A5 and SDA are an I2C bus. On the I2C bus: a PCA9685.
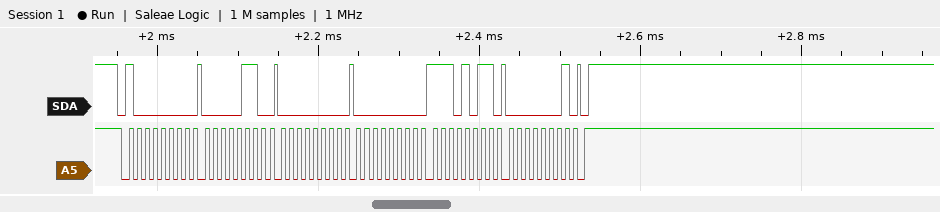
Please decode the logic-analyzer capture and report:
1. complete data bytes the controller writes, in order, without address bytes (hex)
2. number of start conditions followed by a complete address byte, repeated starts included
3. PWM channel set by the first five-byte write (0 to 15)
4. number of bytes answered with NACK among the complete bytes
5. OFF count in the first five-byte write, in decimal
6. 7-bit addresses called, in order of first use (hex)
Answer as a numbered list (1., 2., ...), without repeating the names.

1. 06 00 00 EB 01
2. 1
3. 0
4. 0
5. 491
6. 0x40
